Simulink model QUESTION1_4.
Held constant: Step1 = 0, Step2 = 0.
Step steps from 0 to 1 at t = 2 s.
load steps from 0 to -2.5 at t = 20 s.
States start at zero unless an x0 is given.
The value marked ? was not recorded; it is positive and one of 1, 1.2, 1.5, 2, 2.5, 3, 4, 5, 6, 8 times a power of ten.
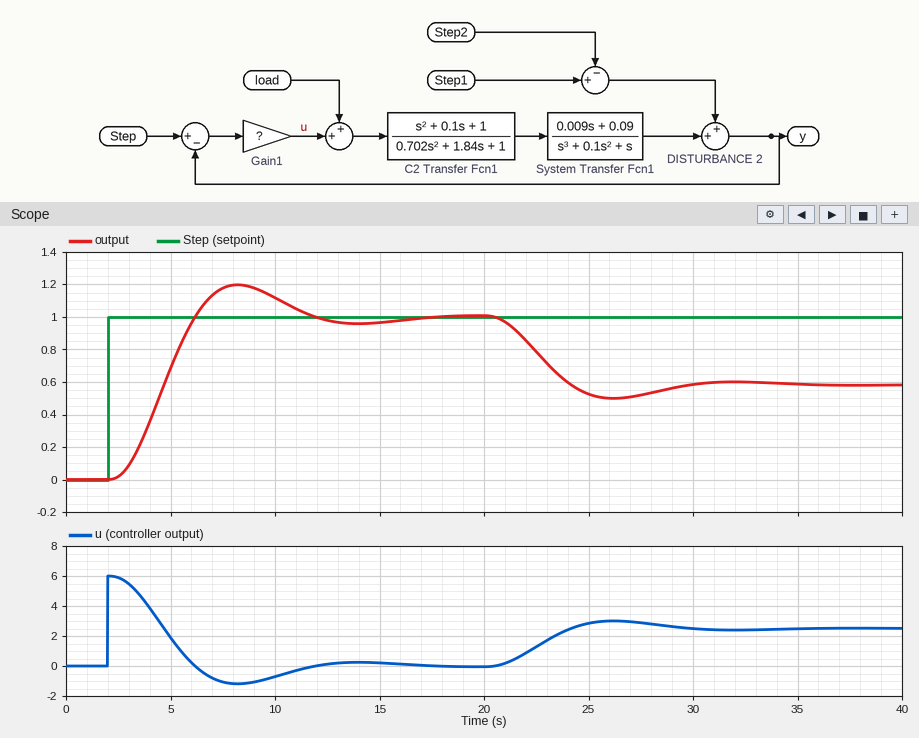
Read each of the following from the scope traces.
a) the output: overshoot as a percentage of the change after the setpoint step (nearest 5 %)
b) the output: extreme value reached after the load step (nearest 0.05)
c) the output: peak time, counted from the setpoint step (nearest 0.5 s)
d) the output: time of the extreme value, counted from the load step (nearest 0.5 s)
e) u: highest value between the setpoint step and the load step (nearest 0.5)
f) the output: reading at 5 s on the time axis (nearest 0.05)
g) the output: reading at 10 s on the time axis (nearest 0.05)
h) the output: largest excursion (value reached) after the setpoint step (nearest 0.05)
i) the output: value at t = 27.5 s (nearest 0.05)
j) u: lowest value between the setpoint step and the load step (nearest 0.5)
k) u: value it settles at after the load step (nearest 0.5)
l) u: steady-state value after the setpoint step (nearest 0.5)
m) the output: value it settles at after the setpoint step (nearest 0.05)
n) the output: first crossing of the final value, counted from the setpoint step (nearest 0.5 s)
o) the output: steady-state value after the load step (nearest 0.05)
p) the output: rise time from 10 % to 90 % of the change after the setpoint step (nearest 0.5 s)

20 %
0.50
6.0 s
6.0 s
6.0
0.70
1.10
1.20
0.50
-1.0
2.5
0.0
1.00
4.0 s
0.60
2.5 s
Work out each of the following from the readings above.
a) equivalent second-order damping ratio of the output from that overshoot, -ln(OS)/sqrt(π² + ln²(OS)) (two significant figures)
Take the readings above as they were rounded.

0.46
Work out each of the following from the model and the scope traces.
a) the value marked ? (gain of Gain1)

6
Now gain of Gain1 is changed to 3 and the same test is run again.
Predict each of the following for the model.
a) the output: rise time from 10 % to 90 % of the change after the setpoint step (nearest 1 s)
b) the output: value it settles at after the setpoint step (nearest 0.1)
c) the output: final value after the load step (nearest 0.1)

5 s
1.0
0.2
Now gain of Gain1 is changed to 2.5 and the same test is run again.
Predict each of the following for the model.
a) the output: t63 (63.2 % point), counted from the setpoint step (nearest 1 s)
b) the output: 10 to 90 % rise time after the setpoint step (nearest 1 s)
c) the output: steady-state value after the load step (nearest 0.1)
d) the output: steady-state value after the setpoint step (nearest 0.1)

5 s
6 s
0.0
1.0
